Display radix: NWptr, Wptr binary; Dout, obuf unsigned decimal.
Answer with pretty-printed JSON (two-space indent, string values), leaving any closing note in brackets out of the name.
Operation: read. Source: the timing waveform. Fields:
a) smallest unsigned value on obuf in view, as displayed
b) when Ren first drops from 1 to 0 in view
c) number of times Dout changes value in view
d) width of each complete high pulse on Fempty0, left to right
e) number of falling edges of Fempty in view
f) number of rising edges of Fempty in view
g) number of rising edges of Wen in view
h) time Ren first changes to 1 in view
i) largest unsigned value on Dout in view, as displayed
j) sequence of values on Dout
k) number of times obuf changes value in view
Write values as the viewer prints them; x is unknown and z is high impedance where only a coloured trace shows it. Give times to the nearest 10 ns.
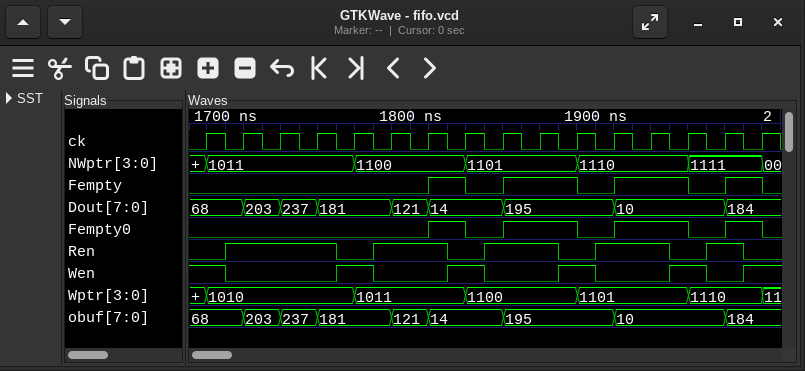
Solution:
{
  "smallest unsigned value on obuf in view, as displayed": "10",
  "when Ren first drops from 1 to 0 in view": "1760 ns",
  "number of times Dout changes value in view": "8",
  "width of each complete high pulse on Fempty0, left to right": "20 ns, 40 ns, 40 ns, 20 ns",
  "number of falling edges of Fempty in view": "4",
  "number of rising edges of Fempty in view": "4",
  "number of rising edges of Wen in view": "5",
  "time Ren first changes to 1 in view": "1700 ns",
  "largest unsigned value on Dout in view, as displayed": "237",
  "sequence of values on Dout": "68, 203, 237, 181, 121, 14, 195, 10, 184",
  "number of times obuf changes value in view": "8"
}
